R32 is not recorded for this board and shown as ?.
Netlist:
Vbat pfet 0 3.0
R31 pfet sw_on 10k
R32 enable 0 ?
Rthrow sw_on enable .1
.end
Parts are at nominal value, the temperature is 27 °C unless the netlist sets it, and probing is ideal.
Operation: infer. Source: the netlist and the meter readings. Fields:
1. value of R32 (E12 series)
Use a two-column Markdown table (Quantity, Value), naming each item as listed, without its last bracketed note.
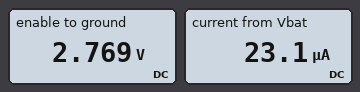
| Quantity | Value |
|---|---|
| value of R32 | 120 kΩ |
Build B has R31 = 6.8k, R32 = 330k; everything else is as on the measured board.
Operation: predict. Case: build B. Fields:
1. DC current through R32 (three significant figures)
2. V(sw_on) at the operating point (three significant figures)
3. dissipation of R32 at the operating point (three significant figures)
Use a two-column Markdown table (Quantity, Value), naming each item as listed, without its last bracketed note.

| Quantity | Value |
|---|---|
| DC current through R32 | 8.91 µA |
| V(sw_on) at the operating point | 2.94 V |
| dissipation of R32 at the operating point | 26.2 µW |
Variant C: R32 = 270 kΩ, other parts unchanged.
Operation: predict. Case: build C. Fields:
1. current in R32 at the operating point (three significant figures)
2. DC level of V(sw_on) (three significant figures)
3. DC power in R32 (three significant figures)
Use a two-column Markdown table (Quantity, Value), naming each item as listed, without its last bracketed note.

| Quantity | Value |
|---|---|
| current in R32 at the operating point | 10.7 µA |
| DC level of V(sw_on) | 2.89 V |
| DC power in R32 | 31.0 µW |
